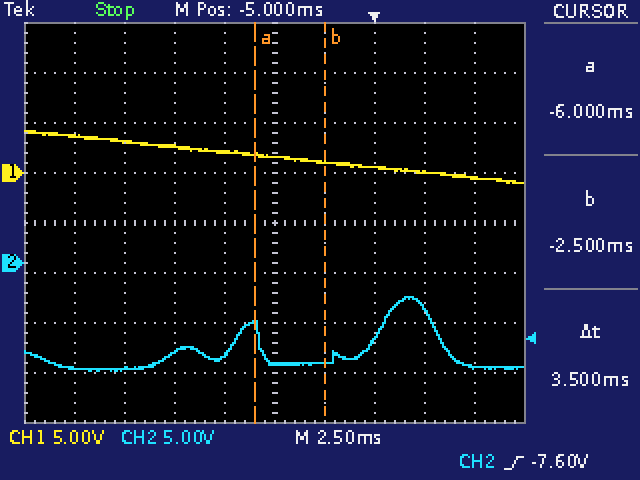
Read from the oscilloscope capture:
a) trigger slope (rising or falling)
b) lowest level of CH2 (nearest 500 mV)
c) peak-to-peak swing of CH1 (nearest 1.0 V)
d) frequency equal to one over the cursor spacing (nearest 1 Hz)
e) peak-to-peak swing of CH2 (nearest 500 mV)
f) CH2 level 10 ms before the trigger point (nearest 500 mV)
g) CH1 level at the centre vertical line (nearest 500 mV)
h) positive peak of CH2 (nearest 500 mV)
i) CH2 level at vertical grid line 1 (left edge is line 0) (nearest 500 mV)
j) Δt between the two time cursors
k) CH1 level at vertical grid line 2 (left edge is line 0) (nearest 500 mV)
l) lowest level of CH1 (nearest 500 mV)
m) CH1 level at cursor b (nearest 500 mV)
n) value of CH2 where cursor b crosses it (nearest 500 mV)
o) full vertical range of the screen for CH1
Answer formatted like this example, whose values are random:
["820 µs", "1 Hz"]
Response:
["rising", "-11.0 V", "5.0 V", "286 Hz", "7.5 V", "-9.0 V", "1.5 V", "-3.5 V", "-10.5 V", "3.5 ms", "3.0 V", "-1.0 V", "1.0 V", "-10.0 V", "40 V"]
